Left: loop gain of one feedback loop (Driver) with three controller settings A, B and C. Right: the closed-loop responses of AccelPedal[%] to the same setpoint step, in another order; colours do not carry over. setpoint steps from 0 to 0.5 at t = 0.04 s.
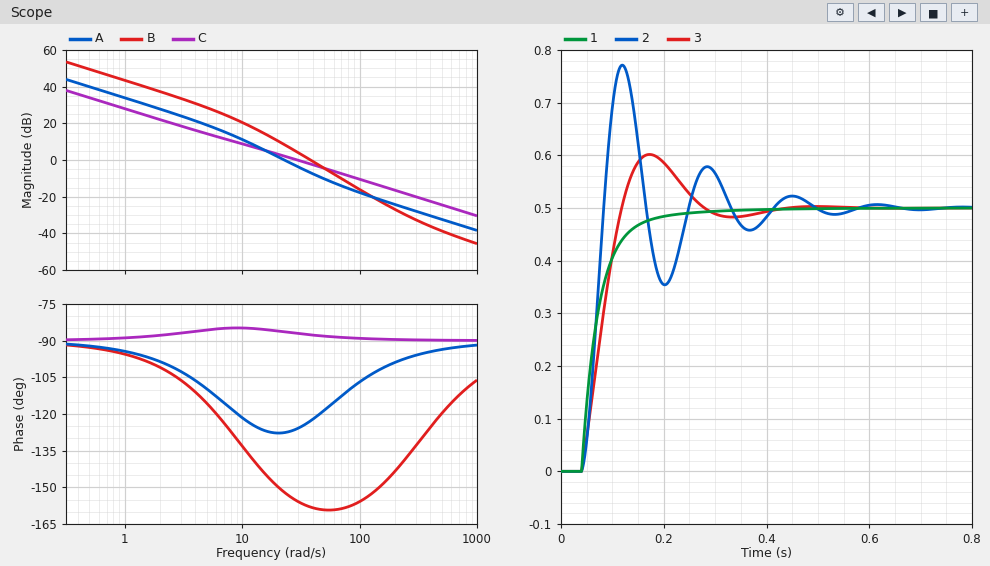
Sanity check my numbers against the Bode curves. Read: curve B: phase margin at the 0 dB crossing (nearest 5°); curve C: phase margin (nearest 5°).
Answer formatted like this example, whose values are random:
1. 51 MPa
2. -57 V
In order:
1. 20°
2. 95°
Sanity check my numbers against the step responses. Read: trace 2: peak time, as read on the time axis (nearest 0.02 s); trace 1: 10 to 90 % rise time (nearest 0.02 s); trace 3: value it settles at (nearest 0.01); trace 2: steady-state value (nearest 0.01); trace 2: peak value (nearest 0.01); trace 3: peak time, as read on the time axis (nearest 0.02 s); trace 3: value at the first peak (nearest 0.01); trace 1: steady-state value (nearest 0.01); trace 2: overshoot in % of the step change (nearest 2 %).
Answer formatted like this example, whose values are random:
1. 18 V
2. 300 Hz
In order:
1. 0.12 s
2. 0.08 s
3. 0.50
4. 0.50
5. 0.77
6. 0.18 s
7. 0.60
8. 0.50
9. 54 %
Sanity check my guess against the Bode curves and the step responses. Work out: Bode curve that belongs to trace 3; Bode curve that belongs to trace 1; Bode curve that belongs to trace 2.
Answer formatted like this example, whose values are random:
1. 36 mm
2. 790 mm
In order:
1. A
2. C
3. B
